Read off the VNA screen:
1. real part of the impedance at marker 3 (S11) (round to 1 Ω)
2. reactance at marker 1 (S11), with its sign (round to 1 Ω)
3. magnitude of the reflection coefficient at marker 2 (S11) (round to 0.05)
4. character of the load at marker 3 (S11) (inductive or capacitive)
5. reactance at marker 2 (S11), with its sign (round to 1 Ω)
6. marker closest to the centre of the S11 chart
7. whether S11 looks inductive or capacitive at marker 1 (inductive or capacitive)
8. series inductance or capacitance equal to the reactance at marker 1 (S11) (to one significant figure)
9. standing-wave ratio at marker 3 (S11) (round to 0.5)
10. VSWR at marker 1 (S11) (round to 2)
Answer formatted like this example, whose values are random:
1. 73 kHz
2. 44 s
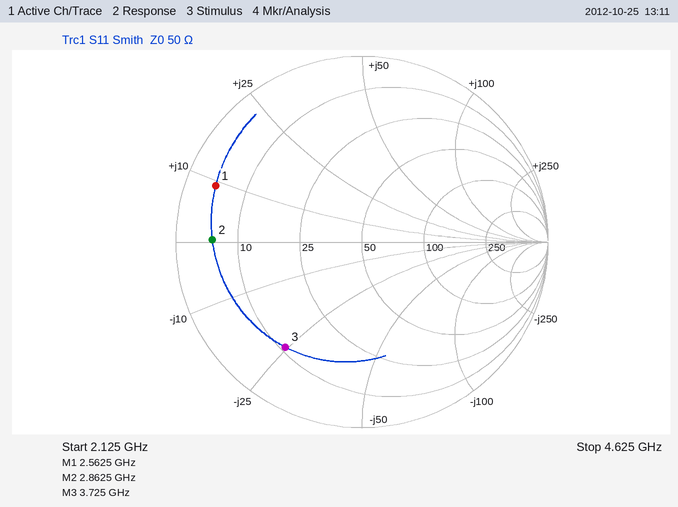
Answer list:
1. 11 Ω
2. +9 Ω
3. 0.80
4. capacitive
5. 0 Ω
6. marker 3
7. inductive
8. 600 pH
9. 5.5
10. 12
